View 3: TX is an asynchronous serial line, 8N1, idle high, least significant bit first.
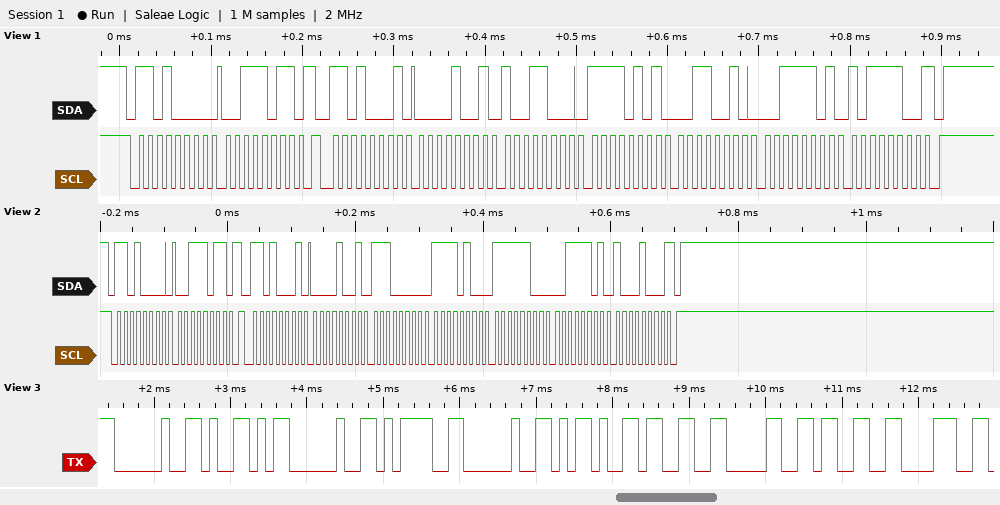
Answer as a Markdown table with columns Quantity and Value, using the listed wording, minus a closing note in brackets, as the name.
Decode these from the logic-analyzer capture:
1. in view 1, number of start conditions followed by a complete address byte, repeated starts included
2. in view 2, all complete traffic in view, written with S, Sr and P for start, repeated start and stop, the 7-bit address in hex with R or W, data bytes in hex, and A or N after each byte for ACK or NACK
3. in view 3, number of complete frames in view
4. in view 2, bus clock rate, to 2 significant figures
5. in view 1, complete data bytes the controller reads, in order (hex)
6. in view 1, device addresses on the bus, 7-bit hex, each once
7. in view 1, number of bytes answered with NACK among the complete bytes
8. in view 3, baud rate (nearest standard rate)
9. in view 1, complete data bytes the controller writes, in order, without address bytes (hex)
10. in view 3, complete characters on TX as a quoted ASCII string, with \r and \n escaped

| Quantity | Value |
|---|---|
| in view 1, number of start conditions followed by a complete address byte, repeated starts included | 2 |
| in view 2, all complete traffic in view, written with S, Sr and P for start, repeated start and stop, the 7-bit address in hex with R or W, data bytes in hex, and A or N after each byte for ACK or NACK | S 68W A 3B A Sr 68R A 09 A E0 A F4 A FC A 3D A 88 N P |
| in view 3, number of complete frames in view | 10 |
| in view 2, bus clock rate, to 2 significant figures | 100 kHz |
| in view 1, complete data bytes the controller reads, in order | 09 98 F5 32 3D BC |
| in view 1, device addresses on the bus, 7-bit hex, each once | 0x68 |
| in view 1, number of bytes answered with NACK among the complete bytes | 1 |
| in view 3, baud rate | 9600 baud |
| in view 1, complete data bytes the controller writes, in order, without address bytes | 3B |
| in view 3, complete characters on TX as a quoted ASCII string, with \r and \n escaped | " Y = -3038" |
